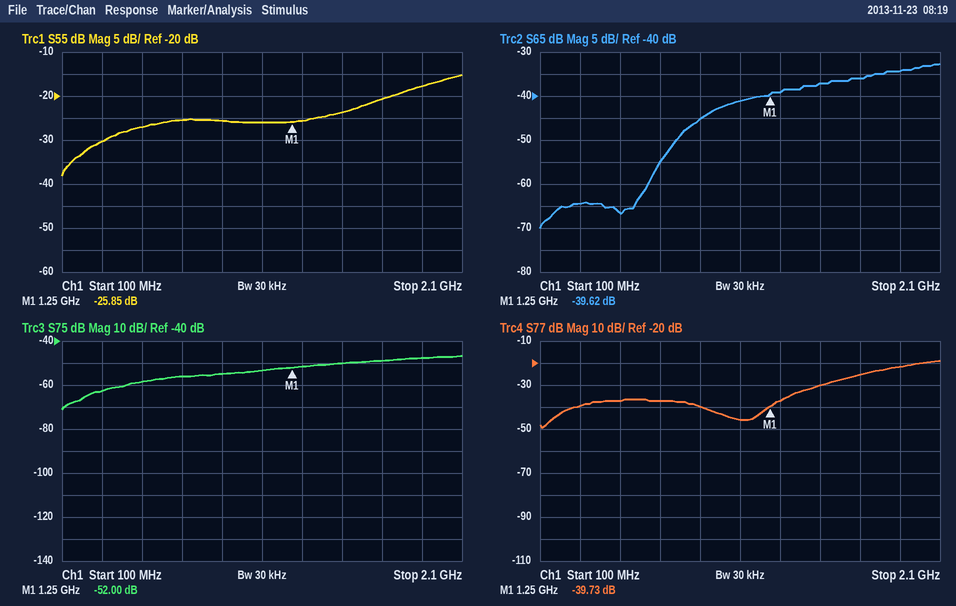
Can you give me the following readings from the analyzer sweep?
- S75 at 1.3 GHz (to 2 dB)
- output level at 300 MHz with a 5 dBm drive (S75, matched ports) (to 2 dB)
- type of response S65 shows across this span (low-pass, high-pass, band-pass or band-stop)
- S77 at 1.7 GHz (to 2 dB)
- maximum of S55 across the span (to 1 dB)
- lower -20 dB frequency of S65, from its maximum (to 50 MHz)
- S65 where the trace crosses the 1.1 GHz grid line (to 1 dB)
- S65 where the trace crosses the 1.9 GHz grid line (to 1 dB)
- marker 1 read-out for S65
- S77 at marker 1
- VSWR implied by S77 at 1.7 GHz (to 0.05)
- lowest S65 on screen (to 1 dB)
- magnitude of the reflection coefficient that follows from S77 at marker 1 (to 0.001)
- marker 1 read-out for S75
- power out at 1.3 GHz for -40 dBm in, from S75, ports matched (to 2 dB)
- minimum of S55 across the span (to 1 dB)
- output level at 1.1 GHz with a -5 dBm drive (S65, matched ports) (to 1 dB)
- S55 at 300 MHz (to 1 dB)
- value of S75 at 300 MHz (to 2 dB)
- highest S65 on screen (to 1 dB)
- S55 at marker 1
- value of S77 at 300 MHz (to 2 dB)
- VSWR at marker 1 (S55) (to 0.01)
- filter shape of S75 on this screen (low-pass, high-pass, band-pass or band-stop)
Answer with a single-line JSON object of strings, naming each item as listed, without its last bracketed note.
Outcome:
{"S75 at 1.3 GHz": "-52 dB", "output level at 300 MHz with a 5 dBm drive (S75, matched ports)": "-58 dBm", "type of response S65 shows across this span": "high-pass", "S77 at 1.7 GHz": "-26 dB", "maximum of S55 across the span": "-15 dB", "lower -20 dB frequency of S65, from its maximum": "750 MHz", "S65 where the trace crosses the 1.1 GHz grid line": "-41 dB", "S65 where the trace crosses the 1.9 GHz grid line": "-34 dB", "marker 1 read-out for S65": "-39.62 dB", "S77 at marker 1": "-39.73 dB", "VSWR implied by S77 at 1.7 GHz": "1.10", "lowest S65 on screen": "-70 dB", "magnitude of the reflection coefficient that follows from S77 at marker 1": "0.010", "marker 1 read-out for S75": "-52.00 dB", "power out at 1.3 GHz for -40 dBm in, from S75, ports matched": "-92 dBm", "minimum of S55 across the span": "-38 dB", "output level at 1.1 GHz with a -5 dBm drive (S65, matched ports)": "-46 dBm", "S55 at 300 MHz": "-30 dB", "value of S75 at 300 MHz": "-62 dB", "highest S65 on screen": "-33 dB", "S55 at marker 1": "-25.85 dB", "value of S77 at 300 MHz": "-40 dB", "VSWR at marker 1 (S55)": "1.11", "filter shape of S75 on this screen": "high-pass"}
